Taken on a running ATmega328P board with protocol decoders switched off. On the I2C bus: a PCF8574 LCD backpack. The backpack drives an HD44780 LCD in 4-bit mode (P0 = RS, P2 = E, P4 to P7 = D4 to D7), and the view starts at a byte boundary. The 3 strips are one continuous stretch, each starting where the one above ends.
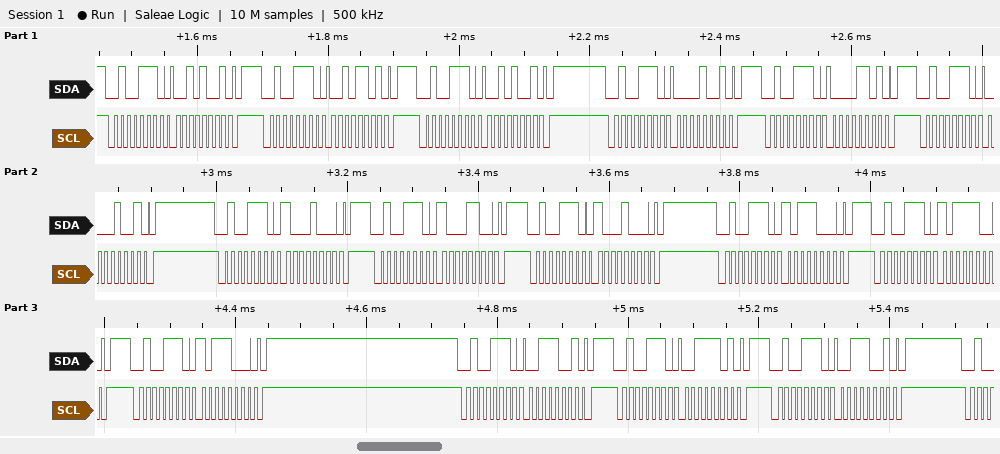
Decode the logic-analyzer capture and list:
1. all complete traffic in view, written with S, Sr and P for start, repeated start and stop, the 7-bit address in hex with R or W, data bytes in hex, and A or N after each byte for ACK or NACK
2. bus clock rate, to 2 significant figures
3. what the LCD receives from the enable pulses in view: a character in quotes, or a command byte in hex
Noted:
S 27W A 29 A P S 27W A 2D A P S 27W A 29 A P S 27W A 09 A P S 27W A 0D A P S 27W A 09 A P S 27W A 88 A P S 27W A 8C A P S 27W A 88 A P S 27W A B8 A P S 27W A BC A P S 27W A B8 A P S 27W A 39 A P S 27W A 3D A P S 27W A 39 A P
100 kHz
' ' 0x8B
